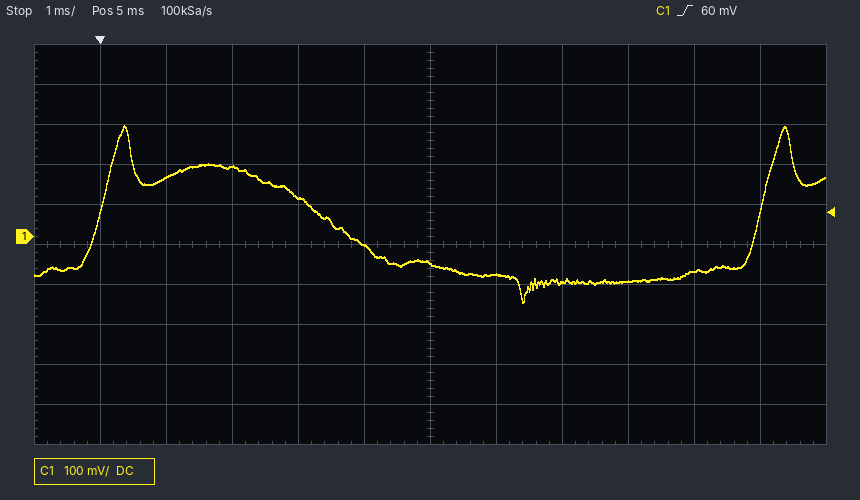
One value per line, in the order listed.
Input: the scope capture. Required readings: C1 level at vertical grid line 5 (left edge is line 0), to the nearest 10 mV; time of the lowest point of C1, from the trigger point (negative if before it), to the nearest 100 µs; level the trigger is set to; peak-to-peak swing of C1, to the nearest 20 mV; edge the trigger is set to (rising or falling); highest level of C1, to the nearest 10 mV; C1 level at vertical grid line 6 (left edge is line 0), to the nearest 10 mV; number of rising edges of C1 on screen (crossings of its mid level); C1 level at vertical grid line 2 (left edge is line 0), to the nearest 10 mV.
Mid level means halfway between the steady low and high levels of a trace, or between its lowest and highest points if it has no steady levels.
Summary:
-20 mV
+6.4 ms
60 mV
440 mV
rising
280 mV
-70 mV
2
150 mV
